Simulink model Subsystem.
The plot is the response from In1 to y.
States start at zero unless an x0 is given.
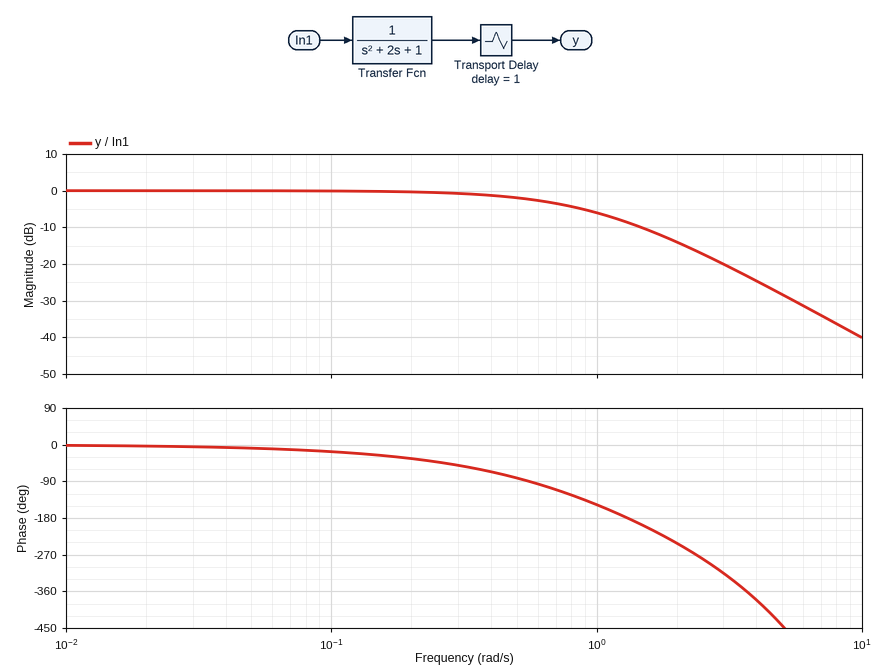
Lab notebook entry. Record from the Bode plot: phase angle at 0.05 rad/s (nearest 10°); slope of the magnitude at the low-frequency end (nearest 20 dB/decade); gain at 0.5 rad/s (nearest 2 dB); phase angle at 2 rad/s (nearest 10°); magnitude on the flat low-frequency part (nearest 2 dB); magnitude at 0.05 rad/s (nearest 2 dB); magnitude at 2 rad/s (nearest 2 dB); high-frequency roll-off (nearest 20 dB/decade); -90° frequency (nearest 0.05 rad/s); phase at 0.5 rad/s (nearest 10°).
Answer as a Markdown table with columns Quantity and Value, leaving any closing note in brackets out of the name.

| Quantity | Value |
|---|---|
| phase angle at 0.05 rad/s | -10° |
| slope of the magnitude at the low-frequency end | 0 dB/decade |
| gain at 0.5 rad/s | -2 dB |
| phase angle at 2 rad/s | -240° |
| magnitude on the flat low-frequency part | 0 dB |
| magnitude at 0.05 rad/s | 0 dB |
| magnitude at 2 rad/s | -14 dB |
| high-frequency roll-off | -40 dB/decade |
| -90° frequency | 0.55 rad/s |
| phase at 0.5 rad/s | -80° |
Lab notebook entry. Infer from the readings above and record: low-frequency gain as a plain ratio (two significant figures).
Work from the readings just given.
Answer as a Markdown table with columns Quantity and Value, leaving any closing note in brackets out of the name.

| Quantity | Value |
|---|---|
| low-frequency gain as a plain ratio | 1.0 |
